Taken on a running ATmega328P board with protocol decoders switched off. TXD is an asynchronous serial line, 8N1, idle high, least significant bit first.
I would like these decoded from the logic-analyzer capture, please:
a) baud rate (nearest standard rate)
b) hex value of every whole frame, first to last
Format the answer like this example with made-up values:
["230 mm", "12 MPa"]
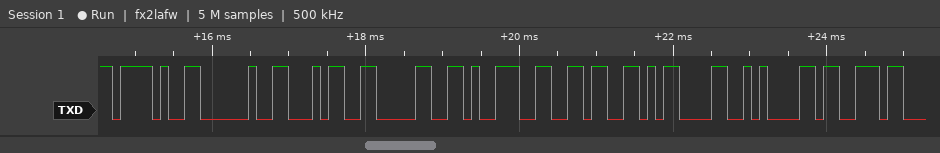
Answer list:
["9600 baud", "0x2F 0x20 0x34 0x30 0x39 0x36 0x0D 0x0A 0x73"]
